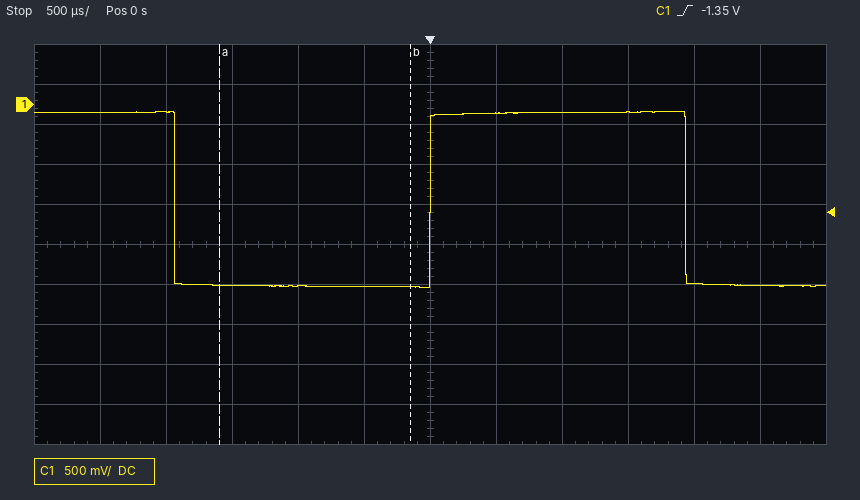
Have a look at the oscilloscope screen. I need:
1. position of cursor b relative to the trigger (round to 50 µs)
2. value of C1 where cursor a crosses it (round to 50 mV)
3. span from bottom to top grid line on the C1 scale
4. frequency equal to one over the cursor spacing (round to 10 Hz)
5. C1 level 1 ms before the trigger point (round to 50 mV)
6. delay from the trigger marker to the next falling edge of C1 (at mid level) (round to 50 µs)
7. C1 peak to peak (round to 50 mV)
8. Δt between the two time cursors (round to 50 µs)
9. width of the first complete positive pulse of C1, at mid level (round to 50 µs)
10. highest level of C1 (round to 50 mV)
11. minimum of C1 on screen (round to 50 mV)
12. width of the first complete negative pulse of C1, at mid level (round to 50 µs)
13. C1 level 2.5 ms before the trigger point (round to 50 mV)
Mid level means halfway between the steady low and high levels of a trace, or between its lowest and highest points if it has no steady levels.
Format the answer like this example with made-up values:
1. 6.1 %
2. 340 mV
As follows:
1. -150 µs
2. -2.25 V
3. 5 V
4. 690 Hz
5. -2.25 V
6. 1.95 ms
7. 2.20 V
8. 1.45 ms
9. 1.95 ms
10. -100 mV
11. -2.30 V
12. 1.95 ms
13. -100 mV
